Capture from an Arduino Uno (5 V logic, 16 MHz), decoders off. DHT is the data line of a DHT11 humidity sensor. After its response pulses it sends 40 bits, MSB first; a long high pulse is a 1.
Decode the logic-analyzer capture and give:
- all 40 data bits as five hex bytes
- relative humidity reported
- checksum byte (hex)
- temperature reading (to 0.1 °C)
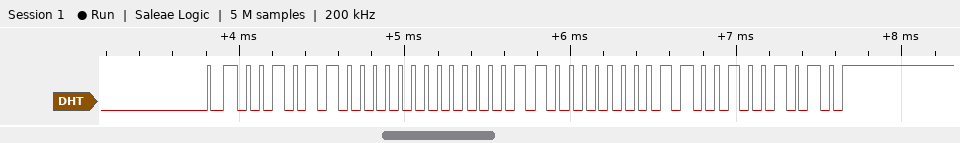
2C 00 18 06 4A
44 %
0x4A
24.6 °C
